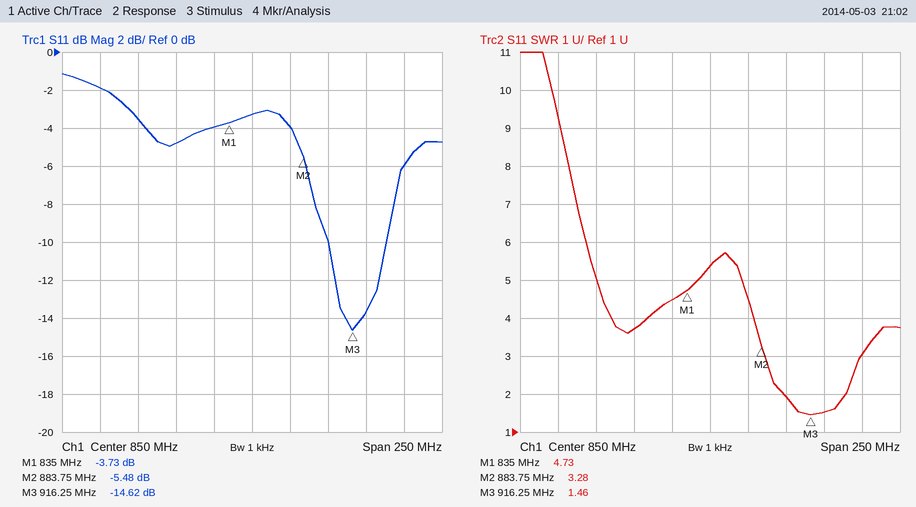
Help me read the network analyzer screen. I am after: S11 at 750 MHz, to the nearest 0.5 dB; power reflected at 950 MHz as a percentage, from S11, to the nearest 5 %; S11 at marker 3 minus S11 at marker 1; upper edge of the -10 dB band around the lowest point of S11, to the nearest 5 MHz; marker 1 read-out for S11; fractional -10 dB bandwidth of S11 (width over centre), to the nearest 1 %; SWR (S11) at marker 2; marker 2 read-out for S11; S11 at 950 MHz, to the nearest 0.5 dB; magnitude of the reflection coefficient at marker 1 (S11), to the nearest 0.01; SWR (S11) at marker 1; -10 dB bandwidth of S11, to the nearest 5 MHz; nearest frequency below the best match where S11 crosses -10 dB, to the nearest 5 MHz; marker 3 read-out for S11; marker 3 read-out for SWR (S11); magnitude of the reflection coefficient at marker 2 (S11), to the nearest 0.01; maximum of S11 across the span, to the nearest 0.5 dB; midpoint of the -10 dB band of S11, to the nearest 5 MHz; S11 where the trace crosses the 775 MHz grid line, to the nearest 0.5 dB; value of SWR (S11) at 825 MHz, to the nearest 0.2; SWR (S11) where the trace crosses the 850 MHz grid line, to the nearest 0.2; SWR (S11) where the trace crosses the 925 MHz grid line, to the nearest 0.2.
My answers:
-2.0 dB
25 %
-10.89 dB
940 MHz
-3.73 dB
4 %
3.28
-5.48 dB
-6.0 dB
0.65
4.73
40 MHz
900 MHz
-14.62 dB
1.46
0.53
-1.0 dB
920 MHz
-3.5 dB
4.4
5.4
1.6
